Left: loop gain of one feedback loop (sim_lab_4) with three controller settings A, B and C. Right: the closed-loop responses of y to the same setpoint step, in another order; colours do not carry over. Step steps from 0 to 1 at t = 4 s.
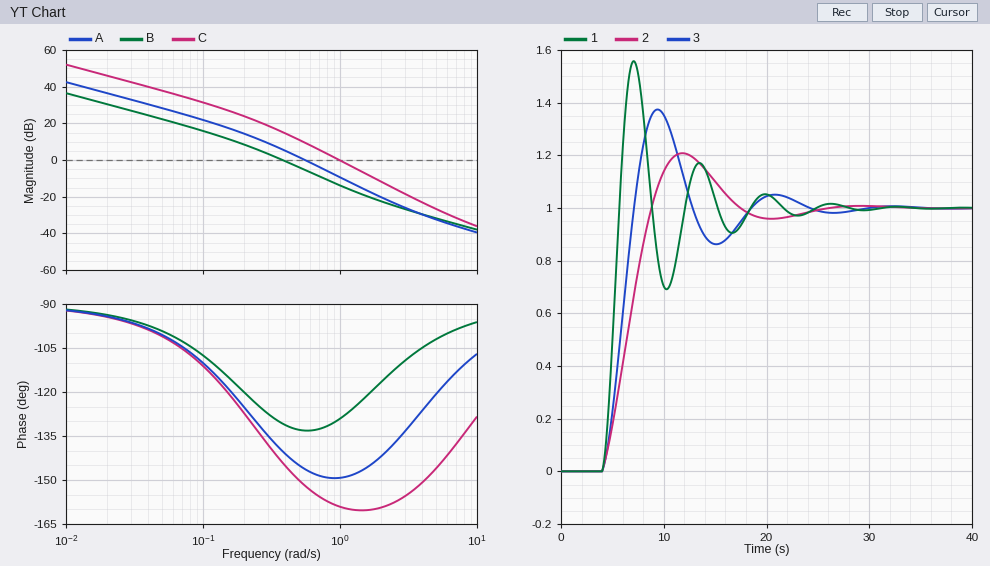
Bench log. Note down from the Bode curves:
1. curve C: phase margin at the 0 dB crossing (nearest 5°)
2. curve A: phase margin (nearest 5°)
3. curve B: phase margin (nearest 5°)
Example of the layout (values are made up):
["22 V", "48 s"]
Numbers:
["20°", "35°", "50°"]
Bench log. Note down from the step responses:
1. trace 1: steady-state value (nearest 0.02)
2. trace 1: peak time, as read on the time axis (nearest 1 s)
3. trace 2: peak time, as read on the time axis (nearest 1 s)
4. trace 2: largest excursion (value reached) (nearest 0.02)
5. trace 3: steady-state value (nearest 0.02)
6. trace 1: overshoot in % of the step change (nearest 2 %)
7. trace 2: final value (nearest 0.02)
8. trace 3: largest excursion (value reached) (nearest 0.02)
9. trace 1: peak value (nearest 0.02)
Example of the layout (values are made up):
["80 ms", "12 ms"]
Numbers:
["1.00", "7 s", "12 s", "1.20", "1.00", "56 %", "1.00", "1.38", "1.56"]
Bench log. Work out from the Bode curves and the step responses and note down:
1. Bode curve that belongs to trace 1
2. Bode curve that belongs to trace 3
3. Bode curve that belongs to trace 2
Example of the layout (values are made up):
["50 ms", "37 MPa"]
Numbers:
["C", "A", "B"]
